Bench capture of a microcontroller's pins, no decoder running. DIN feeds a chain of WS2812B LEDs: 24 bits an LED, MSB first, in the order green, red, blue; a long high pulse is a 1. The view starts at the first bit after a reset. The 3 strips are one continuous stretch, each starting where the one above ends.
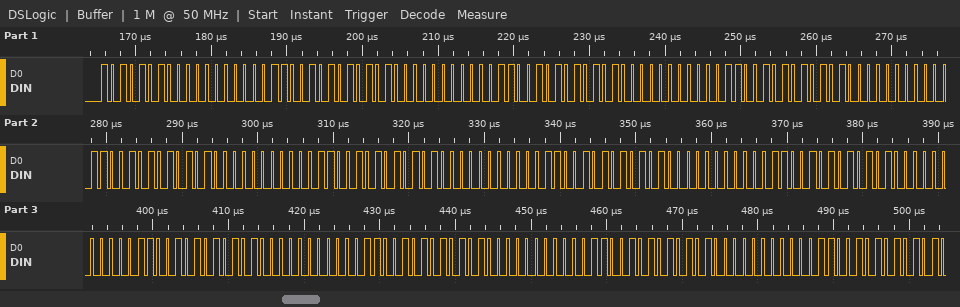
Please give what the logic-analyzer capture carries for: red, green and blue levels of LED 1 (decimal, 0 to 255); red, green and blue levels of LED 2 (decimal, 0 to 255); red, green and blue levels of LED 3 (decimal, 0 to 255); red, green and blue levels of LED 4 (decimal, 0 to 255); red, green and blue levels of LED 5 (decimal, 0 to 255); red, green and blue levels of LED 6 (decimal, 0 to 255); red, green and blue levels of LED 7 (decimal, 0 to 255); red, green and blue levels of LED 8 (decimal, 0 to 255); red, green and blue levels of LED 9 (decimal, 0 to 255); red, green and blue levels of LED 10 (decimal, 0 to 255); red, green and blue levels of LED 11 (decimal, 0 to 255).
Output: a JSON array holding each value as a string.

["0, 170, 50", "0, 170, 50", "0, 170, 50", "0, 170, 50", "0, 170, 50", "0, 170, 50", "0, 170, 50", "0, 170, 50", "0, 170, 50", "0, 170, 50", "0, 170, 50"]
